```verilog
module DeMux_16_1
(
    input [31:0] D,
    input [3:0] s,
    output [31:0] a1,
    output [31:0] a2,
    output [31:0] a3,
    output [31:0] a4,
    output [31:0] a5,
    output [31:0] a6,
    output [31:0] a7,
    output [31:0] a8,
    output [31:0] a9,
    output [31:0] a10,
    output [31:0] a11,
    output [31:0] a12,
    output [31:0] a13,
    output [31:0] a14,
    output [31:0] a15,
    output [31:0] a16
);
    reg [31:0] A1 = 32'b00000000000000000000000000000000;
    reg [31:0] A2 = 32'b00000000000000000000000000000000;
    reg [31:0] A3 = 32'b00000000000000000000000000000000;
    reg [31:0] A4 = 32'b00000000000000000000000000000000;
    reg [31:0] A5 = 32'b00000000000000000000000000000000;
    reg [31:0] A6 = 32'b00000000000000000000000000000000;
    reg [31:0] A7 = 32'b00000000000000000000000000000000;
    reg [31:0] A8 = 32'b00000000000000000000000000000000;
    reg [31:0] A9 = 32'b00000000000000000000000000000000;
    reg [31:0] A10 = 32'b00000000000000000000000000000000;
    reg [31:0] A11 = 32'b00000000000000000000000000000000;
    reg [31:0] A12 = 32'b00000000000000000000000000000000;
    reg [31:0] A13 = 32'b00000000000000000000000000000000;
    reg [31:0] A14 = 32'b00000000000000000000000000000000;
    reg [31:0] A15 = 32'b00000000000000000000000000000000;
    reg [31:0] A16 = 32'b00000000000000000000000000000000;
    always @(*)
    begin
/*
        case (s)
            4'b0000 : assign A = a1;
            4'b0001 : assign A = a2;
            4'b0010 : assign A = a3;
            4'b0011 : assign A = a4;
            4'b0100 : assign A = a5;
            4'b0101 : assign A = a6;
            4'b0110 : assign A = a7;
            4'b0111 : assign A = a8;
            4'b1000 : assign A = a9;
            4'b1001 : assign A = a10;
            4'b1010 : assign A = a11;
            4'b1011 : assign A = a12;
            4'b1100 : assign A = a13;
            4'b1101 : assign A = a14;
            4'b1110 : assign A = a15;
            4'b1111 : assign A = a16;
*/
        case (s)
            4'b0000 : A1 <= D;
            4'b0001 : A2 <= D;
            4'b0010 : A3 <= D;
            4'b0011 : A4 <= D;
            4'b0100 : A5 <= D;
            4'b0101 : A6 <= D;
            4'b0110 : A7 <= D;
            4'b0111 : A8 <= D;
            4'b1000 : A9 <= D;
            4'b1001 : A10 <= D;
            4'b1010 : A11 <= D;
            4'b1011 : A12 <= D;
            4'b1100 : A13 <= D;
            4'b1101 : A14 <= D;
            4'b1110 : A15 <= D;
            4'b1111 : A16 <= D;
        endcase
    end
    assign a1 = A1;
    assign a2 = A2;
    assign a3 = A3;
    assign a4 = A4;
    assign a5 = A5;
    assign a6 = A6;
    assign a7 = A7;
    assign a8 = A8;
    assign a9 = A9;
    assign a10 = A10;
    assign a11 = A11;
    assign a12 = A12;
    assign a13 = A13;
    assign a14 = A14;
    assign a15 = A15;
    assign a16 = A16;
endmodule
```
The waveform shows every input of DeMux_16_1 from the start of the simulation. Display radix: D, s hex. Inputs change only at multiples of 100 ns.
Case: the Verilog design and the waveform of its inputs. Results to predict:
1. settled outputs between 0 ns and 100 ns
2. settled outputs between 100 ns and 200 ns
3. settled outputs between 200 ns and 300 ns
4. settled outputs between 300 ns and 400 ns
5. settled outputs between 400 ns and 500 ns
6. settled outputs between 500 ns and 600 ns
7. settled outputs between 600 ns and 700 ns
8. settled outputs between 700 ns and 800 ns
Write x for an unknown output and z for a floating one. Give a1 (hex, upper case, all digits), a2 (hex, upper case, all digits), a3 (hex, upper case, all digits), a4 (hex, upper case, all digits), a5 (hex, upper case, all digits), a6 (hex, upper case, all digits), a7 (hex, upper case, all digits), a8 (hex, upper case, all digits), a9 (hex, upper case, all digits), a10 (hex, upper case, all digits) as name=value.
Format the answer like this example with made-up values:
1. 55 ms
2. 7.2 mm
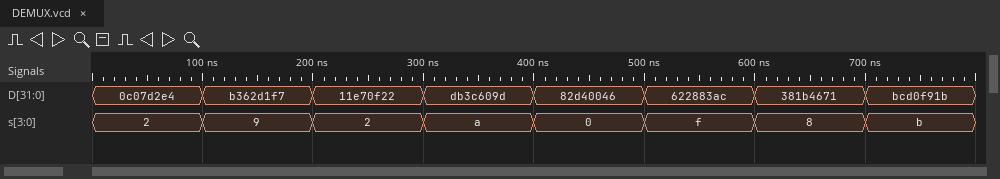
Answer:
1. a1=00000000, a2=00000000, a3=0C07D2E4, a4=00000000, a5=00000000, a6=00000000, a7=00000000, a8=00000000, a9=00000000, a10=00000000
2. a1=00000000, a2=00000000, a3=0C07D2E4, a4=00000000, a5=00000000, a6=00000000, a7=00000000, a8=00000000, a9=00000000, a10=B362D1F7
3. a1=00000000, a2=00000000, a3=11E70F22, a4=00000000, a5=00000000, a6=00000000, a7=00000000, a8=00000000, a9=00000000, a10=B362D1F7
4. a1=00000000, a2=00000000, a3=11E70F22, a4=00000000, a5=00000000, a6=00000000, a7=00000000, a8=00000000, a9=00000000, a10=B362D1F7
5. a1=82D40046, a2=00000000, a3=11E70F22, a4=00000000, a5=00000000, a6=00000000, a7=00000000, a8=00000000, a9=00000000, a10=B362D1F7
6. a1=82D40046, a2=00000000, a3=11E70F22, a4=00000000, a5=00000000, a6=00000000, a7=00000000, a8=00000000, a9=00000000, a10=B362D1F7
7. a1=82D40046, a2=00000000, a3=11E70F22, a4=00000000, a5=00000000, a6=00000000, a7=00000000, a8=00000000, a9=381B4671, a10=B362D1F7
8. a1=82D40046, a2=00000000, a3=11E70F22, a4=00000000, a5=00000000, a6=00000000, a7=00000000, a8=00000000, a9=381B4671, a10=B362D1F7
